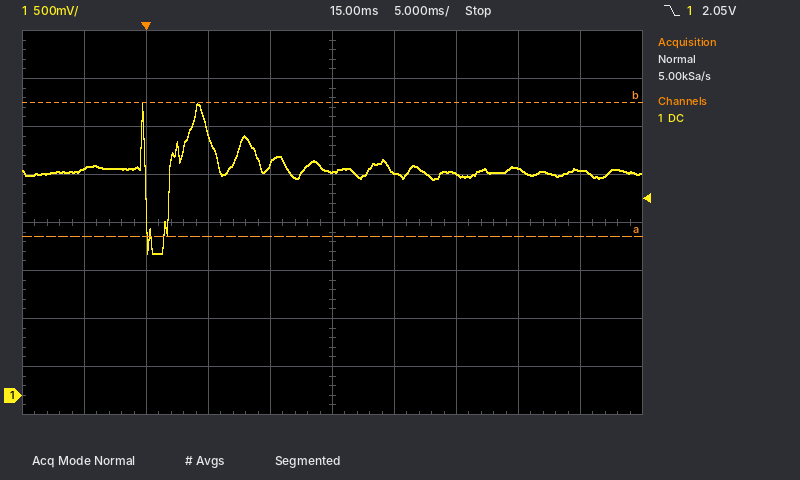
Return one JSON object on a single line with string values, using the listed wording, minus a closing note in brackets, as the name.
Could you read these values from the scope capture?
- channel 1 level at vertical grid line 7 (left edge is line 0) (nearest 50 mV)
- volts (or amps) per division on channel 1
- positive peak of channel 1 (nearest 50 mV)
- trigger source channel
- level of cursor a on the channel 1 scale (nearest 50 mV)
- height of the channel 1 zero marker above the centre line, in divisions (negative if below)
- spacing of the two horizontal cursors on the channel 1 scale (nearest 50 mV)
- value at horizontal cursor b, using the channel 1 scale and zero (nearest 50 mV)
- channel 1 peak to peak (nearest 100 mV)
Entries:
{"channel 1 level at vertical grid line 7 (left edge is line 0)": "2.30 V", "volts (or amps) per division on channel 1": "500 mV", "positive peak of channel 1": "3.05 V", "trigger source channel": "channel 1", "level of cursor a on the channel 1 scale": "1.65 V", "height of the channel 1 zero marker above the centre line, in divisions": "-3.6 div", "spacing of the two horizontal cursors on the channel 1 scale": "1.40 V", "value at horizontal cursor b, using the channel 1 scale and zero": "3.05 V", "channel 1 peak to peak": "1.60 V"}
